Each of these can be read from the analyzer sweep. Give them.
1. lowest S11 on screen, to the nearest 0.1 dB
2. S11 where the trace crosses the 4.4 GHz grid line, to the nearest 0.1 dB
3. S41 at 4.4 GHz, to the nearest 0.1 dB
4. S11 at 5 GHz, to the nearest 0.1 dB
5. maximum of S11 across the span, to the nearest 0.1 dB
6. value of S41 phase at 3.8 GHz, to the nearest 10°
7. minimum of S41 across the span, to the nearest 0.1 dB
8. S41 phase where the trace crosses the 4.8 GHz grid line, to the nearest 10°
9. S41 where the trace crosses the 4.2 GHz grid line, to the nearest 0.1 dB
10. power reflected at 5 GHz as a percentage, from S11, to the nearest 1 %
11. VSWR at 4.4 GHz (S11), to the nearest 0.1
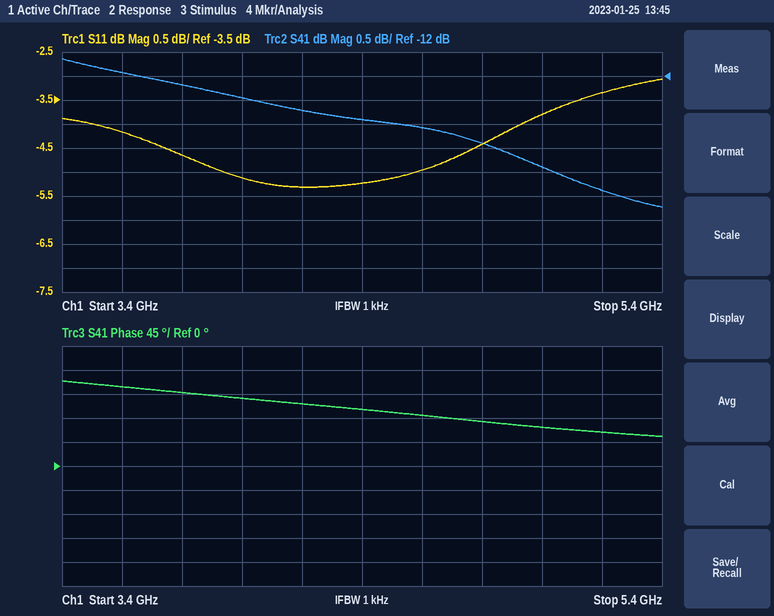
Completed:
-5.3 dB
-5.2 dB
-12.9 dB
-3.8 dB
-3.1 dB
140°
-14.7 dB
80°
-12.7 dB
42 %
3.4
